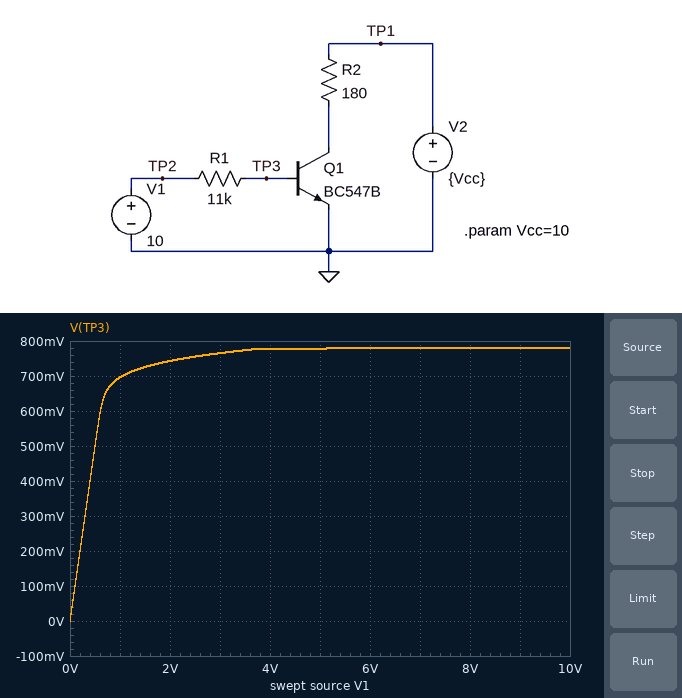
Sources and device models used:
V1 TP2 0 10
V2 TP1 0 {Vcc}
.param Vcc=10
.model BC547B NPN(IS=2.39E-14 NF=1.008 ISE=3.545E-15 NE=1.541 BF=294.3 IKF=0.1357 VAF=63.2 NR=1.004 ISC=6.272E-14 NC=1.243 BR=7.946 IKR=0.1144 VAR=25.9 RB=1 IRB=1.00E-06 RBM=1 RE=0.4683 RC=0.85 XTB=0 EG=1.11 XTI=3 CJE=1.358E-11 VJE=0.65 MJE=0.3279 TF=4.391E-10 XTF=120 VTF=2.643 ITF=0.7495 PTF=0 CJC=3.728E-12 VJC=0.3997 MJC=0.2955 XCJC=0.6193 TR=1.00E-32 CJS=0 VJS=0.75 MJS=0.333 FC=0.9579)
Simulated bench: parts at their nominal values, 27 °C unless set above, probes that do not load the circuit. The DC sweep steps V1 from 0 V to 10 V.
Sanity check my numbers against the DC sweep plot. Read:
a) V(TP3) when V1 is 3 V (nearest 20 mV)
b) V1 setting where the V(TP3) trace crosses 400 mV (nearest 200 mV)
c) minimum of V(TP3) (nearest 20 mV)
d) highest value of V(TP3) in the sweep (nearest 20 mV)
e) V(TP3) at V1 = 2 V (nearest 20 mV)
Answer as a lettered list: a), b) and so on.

a) 760 mV
b) 400 mV
c) 0 V
d) 780 mV
e) 740 mV
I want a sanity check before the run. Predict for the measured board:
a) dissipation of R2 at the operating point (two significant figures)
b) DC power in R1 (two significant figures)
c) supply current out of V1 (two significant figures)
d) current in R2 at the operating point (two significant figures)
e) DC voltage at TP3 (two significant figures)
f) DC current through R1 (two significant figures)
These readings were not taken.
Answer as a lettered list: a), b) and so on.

a) 540 mW
b) 7.7 mW
c) 840 µA
d) 55 mA
e) 780 mV
f) 840 µA
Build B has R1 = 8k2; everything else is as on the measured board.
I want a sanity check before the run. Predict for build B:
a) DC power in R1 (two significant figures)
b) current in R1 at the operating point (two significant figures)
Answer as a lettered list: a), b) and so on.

a) 10 mW
b) 1.1 mA
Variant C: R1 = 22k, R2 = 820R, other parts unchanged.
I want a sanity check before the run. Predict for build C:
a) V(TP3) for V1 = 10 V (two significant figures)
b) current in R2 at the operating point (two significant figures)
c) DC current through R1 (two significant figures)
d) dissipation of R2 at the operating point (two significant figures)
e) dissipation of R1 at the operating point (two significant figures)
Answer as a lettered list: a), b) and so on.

a) 720 mV
b) 12 mA
c) 420 µA
d) 120 mW
e) 3.9 mW
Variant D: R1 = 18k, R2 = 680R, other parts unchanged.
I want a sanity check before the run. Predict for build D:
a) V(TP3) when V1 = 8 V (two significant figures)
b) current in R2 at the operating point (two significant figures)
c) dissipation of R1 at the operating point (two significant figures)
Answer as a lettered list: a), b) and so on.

a) 720 mV
b) 15 mA
c) 4.8 mW
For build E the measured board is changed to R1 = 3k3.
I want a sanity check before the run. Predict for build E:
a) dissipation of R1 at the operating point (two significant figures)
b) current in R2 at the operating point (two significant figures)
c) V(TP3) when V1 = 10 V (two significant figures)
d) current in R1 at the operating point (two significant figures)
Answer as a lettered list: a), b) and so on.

a) 26 mW
b) 55 mA
c) 790 mV
d) 2.8 mA
